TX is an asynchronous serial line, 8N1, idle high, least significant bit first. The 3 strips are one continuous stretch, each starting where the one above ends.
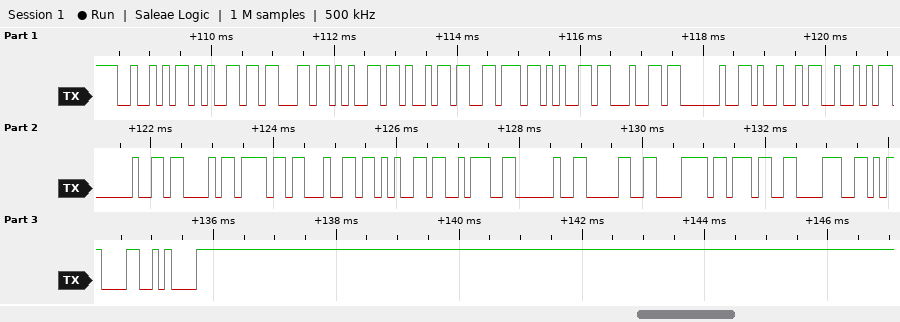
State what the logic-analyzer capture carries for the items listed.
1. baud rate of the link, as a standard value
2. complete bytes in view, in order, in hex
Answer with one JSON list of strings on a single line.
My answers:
["9600 baud", "52 65 63 65 69 76 65 64 20 49 52 20 43 6F 64 65 3A 20 30 78 37 38 0D 0A"]
